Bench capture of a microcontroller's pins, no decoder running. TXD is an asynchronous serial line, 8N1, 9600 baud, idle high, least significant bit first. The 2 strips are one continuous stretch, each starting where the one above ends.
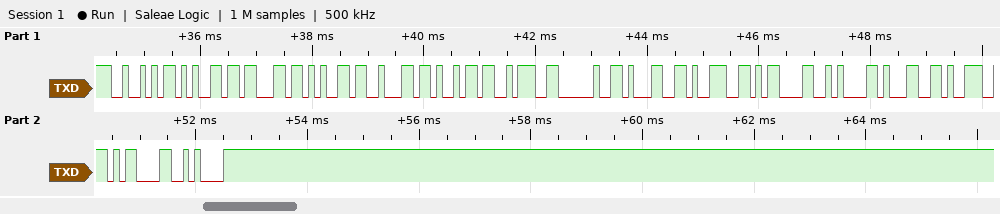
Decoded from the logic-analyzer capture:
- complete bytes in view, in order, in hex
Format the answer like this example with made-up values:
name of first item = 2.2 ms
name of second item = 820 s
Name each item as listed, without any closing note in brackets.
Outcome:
complete bytes in view, in order, in hex = 0x52 0x65 0x63 0x65 0x62 0x69 0x3A 0x20 0x31 0x39 0x0D 0x0A 0x31 0x39 0x0D 0x0A
